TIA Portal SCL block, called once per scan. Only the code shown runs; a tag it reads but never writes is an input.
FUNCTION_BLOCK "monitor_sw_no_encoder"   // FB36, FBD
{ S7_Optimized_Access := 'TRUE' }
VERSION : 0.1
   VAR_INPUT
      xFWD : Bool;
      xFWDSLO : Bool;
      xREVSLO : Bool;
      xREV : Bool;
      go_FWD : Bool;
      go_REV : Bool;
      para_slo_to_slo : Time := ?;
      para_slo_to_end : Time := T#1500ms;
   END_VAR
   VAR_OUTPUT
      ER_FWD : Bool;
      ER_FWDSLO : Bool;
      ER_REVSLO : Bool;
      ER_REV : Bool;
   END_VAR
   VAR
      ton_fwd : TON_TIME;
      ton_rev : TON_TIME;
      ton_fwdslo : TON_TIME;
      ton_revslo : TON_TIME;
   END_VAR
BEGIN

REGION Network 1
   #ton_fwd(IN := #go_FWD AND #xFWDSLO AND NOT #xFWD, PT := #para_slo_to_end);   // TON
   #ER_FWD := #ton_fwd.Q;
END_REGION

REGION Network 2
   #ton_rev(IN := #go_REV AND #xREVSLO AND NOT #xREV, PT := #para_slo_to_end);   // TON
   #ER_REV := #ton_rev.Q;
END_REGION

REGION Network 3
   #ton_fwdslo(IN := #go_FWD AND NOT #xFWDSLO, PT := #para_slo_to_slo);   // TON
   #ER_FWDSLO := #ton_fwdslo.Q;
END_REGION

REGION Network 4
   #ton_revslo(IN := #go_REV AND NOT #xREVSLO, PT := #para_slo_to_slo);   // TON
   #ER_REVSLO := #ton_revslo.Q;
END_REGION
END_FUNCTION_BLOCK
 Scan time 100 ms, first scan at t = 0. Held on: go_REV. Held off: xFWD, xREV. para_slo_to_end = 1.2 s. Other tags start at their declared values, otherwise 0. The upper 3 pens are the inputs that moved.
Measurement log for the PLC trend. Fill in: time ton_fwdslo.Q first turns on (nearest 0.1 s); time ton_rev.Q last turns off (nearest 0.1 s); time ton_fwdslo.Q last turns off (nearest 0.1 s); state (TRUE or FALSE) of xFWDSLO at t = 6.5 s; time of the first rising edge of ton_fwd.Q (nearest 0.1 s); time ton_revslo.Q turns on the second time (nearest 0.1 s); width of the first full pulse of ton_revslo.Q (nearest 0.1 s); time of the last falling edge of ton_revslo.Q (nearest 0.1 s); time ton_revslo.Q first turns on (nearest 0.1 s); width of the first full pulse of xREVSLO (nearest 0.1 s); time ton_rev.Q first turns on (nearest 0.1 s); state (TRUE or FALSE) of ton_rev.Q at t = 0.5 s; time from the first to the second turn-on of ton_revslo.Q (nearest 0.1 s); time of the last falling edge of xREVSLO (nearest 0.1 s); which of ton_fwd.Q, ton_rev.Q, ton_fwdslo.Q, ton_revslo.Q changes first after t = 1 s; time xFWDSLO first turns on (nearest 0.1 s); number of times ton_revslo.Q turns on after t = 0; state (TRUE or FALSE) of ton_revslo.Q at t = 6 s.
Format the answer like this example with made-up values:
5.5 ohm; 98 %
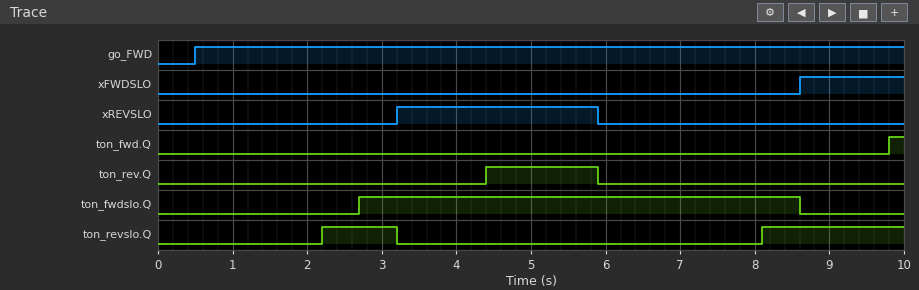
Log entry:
2.7 s; 5.9 s; 8.6 s; FALSE; 9.8 s; 8.1 s; 1.0 s; 3.2 s; 2.2 s; 2.7 s; 4.4 s; FALSE; 5.9 s; 5.9 s; ton_revslo.Q; 8.6 s; 2; FALSE
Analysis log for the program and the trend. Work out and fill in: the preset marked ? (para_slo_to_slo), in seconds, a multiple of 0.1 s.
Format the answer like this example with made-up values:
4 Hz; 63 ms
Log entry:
2.2 s
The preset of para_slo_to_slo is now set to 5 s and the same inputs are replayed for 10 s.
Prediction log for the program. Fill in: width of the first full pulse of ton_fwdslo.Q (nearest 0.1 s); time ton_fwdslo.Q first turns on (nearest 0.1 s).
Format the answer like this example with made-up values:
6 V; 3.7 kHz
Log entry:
3.1 s; 5.5 s
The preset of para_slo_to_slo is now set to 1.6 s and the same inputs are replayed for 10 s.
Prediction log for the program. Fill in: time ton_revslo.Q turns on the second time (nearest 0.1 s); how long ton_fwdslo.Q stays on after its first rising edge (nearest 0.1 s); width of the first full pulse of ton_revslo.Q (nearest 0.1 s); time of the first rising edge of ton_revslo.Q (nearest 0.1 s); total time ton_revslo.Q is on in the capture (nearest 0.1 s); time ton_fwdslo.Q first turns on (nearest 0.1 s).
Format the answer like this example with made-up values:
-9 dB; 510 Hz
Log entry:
7.5 s; 6.5 s; 1.6 s; 1.6 s; 4.1 s; 2.1 s
